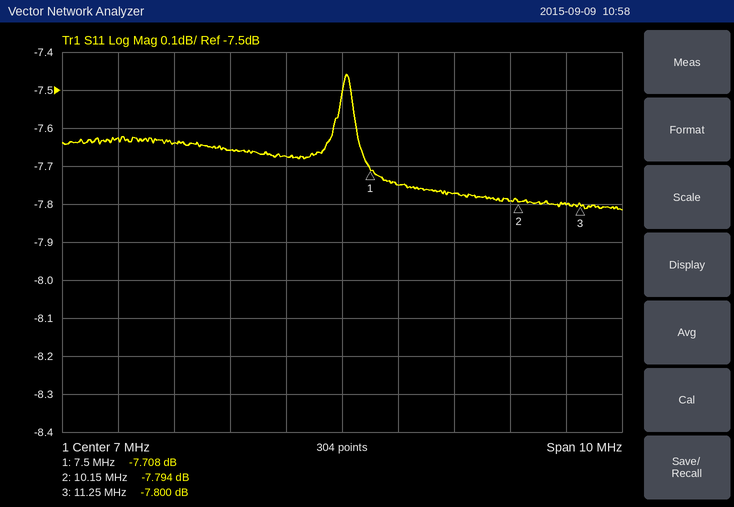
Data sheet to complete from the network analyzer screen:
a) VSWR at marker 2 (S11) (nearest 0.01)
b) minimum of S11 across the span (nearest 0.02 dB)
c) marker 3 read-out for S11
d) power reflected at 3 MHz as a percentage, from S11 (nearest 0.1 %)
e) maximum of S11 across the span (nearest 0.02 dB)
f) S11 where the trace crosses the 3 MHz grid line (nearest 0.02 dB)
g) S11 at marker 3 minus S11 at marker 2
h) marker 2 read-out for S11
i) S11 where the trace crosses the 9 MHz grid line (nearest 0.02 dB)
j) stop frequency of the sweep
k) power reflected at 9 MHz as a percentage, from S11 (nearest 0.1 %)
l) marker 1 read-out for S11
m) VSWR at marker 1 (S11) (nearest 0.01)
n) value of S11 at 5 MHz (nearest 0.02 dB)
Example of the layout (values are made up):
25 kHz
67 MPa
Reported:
2.38
-7.82 dB
-7.800 dB
17.3 %
-7.46 dB
-7.62 dB
-0.006 dB
-7.794 dB
-7.78 dB
12 MHz
16.7 %
-7.708 dB
2.40
-7.66 dB
